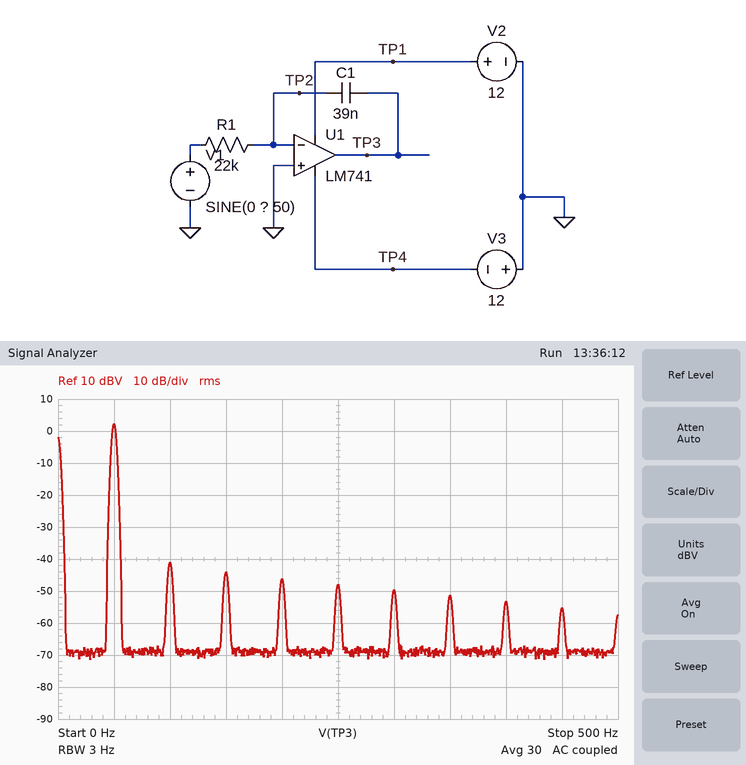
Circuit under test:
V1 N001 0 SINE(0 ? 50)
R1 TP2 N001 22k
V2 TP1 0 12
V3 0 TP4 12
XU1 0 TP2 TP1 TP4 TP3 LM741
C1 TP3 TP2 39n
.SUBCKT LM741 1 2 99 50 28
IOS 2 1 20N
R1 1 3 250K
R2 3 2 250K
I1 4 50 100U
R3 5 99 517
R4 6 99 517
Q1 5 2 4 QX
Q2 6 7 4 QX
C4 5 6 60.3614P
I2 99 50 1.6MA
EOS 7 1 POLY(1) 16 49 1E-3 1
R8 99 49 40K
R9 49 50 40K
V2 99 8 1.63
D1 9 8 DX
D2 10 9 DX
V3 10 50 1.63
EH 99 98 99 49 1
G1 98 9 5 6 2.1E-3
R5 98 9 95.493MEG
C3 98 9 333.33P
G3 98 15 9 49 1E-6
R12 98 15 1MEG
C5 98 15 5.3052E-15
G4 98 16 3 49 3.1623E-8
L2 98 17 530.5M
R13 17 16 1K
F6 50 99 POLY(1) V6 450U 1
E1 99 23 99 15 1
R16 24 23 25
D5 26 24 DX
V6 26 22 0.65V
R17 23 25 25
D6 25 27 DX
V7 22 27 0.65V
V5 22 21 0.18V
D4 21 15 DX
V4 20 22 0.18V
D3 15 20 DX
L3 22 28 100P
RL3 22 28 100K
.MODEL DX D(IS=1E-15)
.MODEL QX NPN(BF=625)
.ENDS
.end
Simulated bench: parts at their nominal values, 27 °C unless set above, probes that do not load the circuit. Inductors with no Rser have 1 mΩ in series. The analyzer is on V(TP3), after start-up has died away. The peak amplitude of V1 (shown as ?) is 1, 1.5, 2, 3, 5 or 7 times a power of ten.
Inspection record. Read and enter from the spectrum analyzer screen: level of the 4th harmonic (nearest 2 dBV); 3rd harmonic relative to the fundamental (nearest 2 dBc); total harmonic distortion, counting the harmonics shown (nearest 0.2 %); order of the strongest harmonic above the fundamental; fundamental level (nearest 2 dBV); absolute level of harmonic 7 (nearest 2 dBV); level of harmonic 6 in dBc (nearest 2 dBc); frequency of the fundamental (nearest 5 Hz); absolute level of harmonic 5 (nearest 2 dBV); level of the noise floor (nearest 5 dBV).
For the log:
-46 dBV
-46 dBc
1.0 %
2
2 dBV
-52 dBV
-52 dBc
50 Hz
-48 dBV
-70 dBV
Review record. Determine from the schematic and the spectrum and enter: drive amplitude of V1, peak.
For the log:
500 mV
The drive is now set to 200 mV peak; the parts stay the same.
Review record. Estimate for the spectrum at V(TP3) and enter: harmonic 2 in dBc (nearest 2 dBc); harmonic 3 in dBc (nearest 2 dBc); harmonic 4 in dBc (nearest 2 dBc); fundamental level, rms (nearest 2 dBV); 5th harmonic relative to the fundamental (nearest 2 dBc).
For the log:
-36 dBc
-40 dBc
-42 dBc
-6 dBV
-46 dBc
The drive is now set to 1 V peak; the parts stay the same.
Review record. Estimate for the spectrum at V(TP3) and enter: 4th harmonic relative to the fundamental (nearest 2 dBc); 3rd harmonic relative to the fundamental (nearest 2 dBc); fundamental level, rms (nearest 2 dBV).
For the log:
-54 dBc
-52 dBc
8 dBV
